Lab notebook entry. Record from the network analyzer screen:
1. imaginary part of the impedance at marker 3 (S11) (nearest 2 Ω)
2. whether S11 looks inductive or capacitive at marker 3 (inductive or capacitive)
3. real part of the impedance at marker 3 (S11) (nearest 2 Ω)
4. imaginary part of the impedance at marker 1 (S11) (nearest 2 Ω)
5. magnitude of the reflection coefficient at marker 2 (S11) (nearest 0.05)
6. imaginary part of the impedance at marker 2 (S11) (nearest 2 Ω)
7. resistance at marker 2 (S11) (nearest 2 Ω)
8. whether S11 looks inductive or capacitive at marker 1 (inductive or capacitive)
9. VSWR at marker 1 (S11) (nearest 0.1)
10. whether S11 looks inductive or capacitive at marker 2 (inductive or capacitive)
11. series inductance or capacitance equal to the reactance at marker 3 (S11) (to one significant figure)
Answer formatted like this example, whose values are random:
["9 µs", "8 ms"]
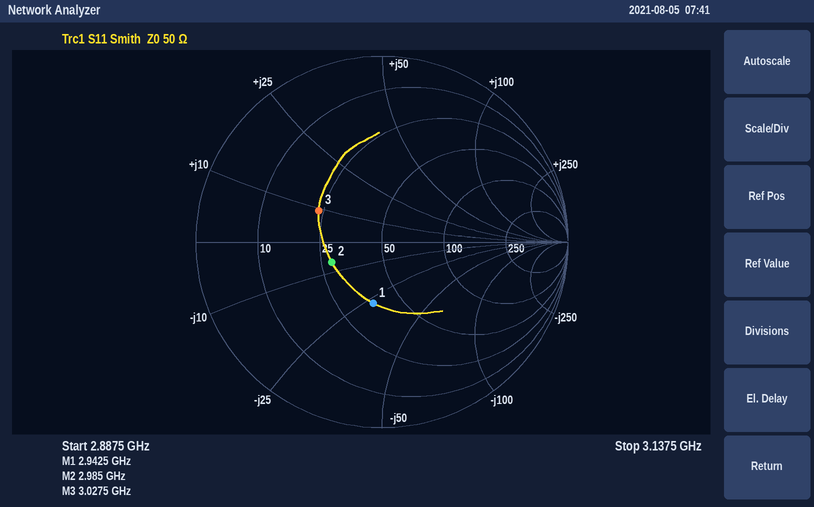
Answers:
["+10 Ω", "inductive", "24 Ω", "-28 Ω", "0.30", "-6 Ω", "28 Ω", "capacitive", "2.0", "capacitive", "500 pH"]
